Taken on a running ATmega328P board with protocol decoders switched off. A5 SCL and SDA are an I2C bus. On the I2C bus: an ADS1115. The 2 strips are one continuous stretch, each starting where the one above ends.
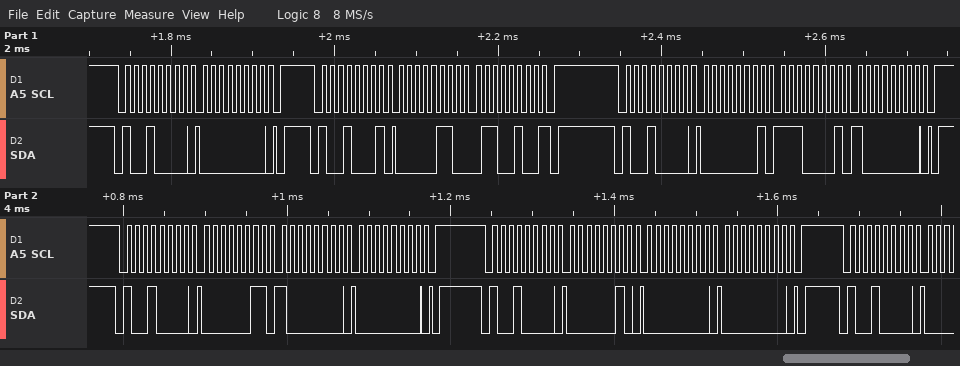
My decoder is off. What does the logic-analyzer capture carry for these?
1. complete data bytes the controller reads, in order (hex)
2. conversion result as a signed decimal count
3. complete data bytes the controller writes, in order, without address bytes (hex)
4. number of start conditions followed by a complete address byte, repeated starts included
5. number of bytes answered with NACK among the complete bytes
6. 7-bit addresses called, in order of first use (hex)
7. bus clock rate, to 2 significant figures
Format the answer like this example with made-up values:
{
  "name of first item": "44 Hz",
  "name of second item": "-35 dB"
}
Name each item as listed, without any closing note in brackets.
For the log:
{
  "complete data bytes the controller reads, in order": "06 64",
  "conversion result as a signed decimal count": "1636",
  "complete data bytes the controller writes, in order, without address bytes": "00 01 E1 80 03 80 00 02 00 00",
  "number of start conditions followed by a complete address byte, repeated starts included": "6",
  "number of bytes answered with NACK among the complete bytes": "1",
  "7-bit addresses called, in order of first use": "0x48",
  "bus clock rate, to 2 significant figures": "100 kHz"
}
